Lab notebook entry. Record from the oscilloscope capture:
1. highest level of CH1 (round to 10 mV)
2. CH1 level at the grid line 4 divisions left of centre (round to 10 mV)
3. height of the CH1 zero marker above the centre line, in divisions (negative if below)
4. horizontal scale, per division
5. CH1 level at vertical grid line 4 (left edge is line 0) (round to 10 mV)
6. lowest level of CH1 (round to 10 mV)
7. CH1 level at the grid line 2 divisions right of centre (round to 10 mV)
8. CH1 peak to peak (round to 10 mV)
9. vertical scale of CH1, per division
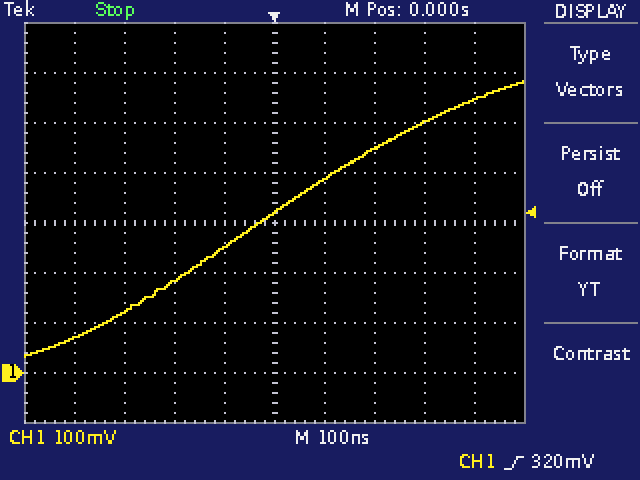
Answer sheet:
580 mV
70 mV
-3.0 div
100 ns
250 mV
30 mV
450 mV
550 mV
100 mV
